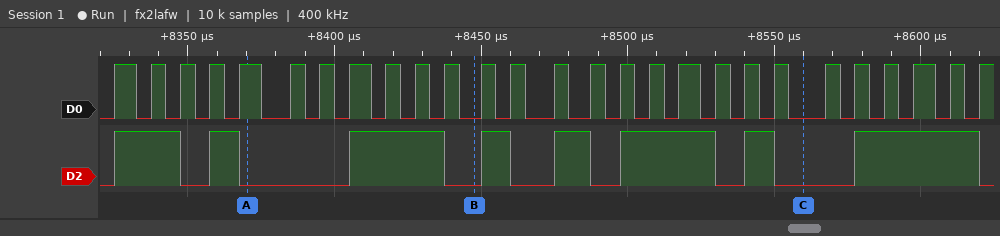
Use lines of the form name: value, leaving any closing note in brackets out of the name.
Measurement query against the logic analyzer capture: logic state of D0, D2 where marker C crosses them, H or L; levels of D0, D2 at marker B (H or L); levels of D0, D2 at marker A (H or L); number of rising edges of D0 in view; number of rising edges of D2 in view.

logic state of D0, D2 where marker C crosses them, H or L: D0=L, D2=L
levels of D0, D2 at marker B: D0=L, D2=L
levels of D0, D2 at marker A: D0=H, D2=L
number of rising edges of D0 in view: 27
number of rising edges of D2 in view: 8
